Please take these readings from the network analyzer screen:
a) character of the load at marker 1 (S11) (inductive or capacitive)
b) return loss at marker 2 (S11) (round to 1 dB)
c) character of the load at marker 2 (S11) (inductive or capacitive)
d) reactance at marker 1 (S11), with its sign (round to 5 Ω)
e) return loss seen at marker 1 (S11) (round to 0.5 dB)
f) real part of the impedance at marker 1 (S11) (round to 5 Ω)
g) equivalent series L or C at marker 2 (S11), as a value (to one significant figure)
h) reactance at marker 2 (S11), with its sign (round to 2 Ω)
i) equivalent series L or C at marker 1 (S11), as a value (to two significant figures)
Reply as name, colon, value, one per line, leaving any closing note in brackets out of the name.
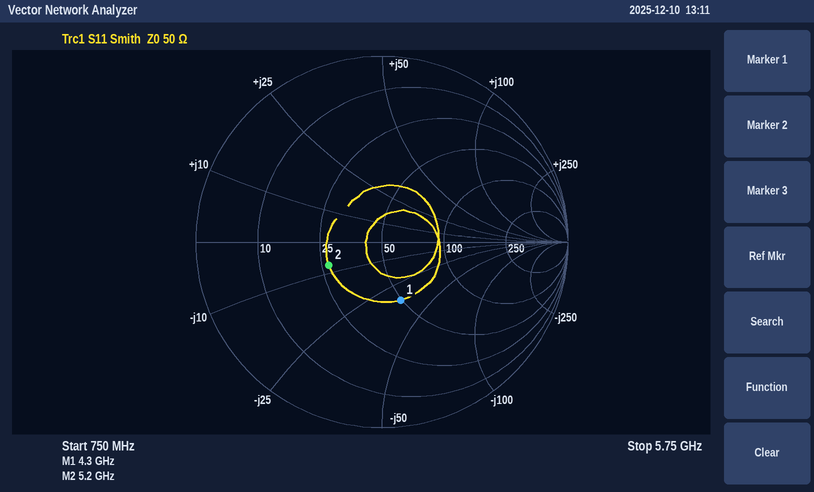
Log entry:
character of the load at marker 1 (S11): capacitive
return loss at marker 2 (S11): 10 dB
character of the load at marker 2 (S11): capacitive
reactance at marker 1 (S11), with its sign: -35 Ω
return loss seen at marker 1 (S11): 9.5 dB
real part of the impedance at marker 1 (S11): 50 Ω
equivalent series L or C at marker 2 (S11), as a value: 4 pF
reactance at marker 2 (S11), with its sign: -8 Ω
equivalent series L or C at marker 1 (S11), as a value: 1.1 pF
